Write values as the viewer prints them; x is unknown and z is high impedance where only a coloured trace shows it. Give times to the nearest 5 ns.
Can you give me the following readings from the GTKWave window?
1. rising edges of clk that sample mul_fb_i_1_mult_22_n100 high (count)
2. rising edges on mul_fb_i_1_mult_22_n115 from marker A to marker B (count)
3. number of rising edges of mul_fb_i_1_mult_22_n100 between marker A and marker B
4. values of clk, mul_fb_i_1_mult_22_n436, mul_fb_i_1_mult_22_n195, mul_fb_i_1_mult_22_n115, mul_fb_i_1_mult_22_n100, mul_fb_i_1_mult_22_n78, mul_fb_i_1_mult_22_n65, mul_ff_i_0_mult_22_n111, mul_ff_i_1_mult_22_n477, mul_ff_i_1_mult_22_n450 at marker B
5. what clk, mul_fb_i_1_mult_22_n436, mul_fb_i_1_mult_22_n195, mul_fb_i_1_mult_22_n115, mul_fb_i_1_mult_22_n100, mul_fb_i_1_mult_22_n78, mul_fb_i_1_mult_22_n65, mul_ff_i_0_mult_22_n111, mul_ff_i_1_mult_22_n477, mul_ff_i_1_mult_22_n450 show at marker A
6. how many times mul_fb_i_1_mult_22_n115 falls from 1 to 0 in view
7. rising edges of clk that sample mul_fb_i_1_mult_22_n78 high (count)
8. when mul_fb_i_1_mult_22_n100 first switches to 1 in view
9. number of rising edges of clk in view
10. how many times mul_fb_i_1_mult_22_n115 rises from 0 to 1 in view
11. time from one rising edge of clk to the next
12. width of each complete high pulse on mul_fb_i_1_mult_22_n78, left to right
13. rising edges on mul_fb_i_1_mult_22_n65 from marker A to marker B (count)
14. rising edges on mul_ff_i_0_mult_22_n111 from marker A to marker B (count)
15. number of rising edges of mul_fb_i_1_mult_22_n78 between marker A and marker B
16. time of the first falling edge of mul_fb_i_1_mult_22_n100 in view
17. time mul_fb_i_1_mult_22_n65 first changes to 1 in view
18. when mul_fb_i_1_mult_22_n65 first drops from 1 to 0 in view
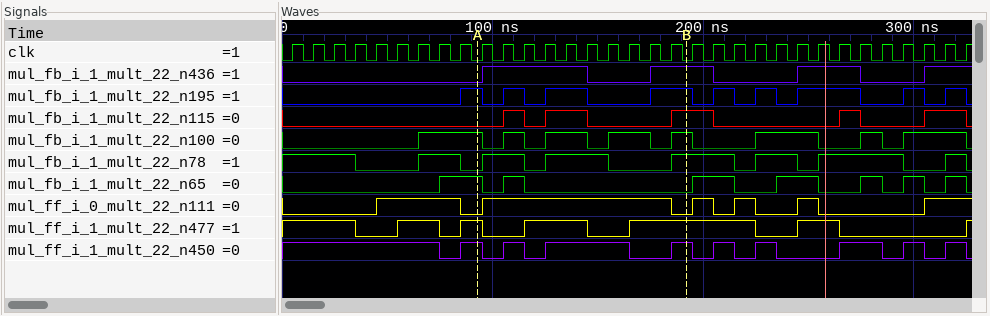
16
3
4
clk=0, mul_fb_i_1_mult_22_n436=1, mul_fb_i_1_mult_22_n195=1, mul_fb_i_1_mult_22_n115=1, mul_fb_i_1_mult_22_n100=1, mul_fb_i_1_mult_22_n78=1, mul_fb_i_1_mult_22_n65=0, mul_ff_i_0_mult_22_n111=0, mul_ff_i_1_mult_22_n477=1, mul_ff_i_1_mult_22_n450=1
clk=0, mul_fb_i_1_mult_22_n436=0, mul_fb_i_1_mult_22_n195=1, mul_fb_i_1_mult_22_n115=0, mul_fb_i_1_mult_22_n100=1, mul_fb_i_1_mult_22_n78=0, mul_fb_i_1_mult_22_n65=1, mul_ff_i_0_mult_22_n111=0, mul_ff_i_1_mult_22_n477=1, mul_ff_i_1_mult_22_n450=1
5
21
65 ns
33
5
10 ns
20 ns, 20 ns, 30 ns, 30 ns, 20 ns, 40 ns, 10 ns
1
1
3
95 ns
75 ns
95 ns
